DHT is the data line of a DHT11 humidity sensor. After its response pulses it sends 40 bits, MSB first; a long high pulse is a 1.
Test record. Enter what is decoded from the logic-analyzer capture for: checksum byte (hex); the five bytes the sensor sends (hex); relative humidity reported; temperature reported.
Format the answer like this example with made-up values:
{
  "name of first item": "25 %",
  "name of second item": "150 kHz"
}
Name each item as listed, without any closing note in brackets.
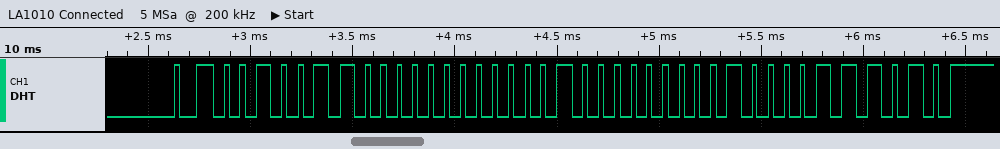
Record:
{
  "checksum byte": "0x3A",
  "the five bytes the sensor sends": "26 00 10 04 3A",
  "relative humidity reported": "38 %",
  "temperature reported": "16.4 °C"
}
